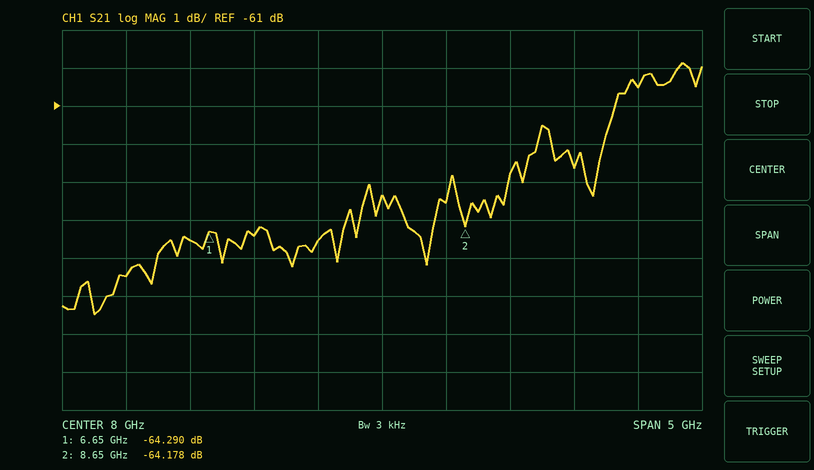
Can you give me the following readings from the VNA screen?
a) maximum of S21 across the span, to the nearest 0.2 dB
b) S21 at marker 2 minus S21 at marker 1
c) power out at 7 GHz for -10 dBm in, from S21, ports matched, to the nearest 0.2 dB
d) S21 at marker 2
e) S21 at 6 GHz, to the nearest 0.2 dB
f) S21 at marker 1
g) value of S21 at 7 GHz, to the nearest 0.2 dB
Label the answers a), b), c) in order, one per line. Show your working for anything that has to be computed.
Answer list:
a) -59.8 dB
b) -64.178 − (-64.29) = 0.112 dB
c) -10 dBm + (-64.4 dB) = -74.4 dBm
d) -64.178 dB
e) -65.4 dB
f) -64.290 dB
g) -64.4 dB
